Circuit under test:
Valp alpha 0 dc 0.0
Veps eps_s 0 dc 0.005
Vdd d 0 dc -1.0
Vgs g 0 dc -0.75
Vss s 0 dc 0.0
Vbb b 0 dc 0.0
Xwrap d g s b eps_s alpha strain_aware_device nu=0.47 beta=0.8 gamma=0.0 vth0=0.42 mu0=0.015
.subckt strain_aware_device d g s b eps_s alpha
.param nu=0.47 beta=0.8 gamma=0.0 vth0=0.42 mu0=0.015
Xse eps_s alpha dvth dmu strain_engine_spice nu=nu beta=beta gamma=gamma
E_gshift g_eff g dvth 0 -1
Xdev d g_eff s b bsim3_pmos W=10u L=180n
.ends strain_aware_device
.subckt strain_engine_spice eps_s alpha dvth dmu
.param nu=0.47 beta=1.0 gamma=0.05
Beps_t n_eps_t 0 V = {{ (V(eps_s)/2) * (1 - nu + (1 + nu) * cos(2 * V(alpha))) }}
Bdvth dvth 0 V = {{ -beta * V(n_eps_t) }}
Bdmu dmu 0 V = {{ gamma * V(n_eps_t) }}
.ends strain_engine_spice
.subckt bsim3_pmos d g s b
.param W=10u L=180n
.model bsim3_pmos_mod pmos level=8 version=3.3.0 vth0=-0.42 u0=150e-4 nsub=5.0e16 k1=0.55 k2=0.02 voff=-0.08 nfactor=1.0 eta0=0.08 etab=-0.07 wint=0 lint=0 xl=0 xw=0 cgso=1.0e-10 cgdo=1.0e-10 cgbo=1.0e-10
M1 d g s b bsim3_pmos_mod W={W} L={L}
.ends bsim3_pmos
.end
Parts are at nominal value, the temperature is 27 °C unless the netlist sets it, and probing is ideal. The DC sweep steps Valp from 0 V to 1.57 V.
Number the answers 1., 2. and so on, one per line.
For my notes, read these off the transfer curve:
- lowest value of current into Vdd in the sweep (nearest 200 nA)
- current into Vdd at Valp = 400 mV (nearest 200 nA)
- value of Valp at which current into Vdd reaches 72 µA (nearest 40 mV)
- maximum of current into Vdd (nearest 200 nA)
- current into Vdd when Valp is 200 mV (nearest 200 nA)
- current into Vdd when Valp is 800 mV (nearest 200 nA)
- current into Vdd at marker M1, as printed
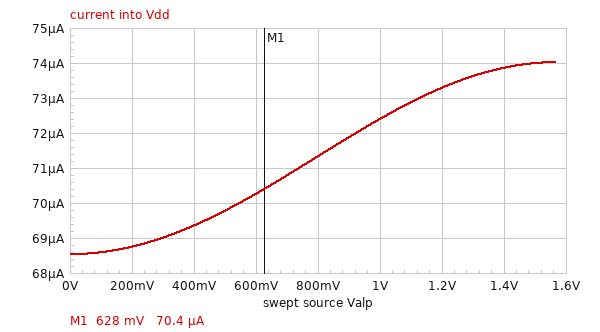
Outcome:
1. 68.6 µA
2. 69.4 µA
3. 920 mV
4. 74.0 µA
5. 68.8 µA
6. 71.4 µA
7. 70.4 µA
